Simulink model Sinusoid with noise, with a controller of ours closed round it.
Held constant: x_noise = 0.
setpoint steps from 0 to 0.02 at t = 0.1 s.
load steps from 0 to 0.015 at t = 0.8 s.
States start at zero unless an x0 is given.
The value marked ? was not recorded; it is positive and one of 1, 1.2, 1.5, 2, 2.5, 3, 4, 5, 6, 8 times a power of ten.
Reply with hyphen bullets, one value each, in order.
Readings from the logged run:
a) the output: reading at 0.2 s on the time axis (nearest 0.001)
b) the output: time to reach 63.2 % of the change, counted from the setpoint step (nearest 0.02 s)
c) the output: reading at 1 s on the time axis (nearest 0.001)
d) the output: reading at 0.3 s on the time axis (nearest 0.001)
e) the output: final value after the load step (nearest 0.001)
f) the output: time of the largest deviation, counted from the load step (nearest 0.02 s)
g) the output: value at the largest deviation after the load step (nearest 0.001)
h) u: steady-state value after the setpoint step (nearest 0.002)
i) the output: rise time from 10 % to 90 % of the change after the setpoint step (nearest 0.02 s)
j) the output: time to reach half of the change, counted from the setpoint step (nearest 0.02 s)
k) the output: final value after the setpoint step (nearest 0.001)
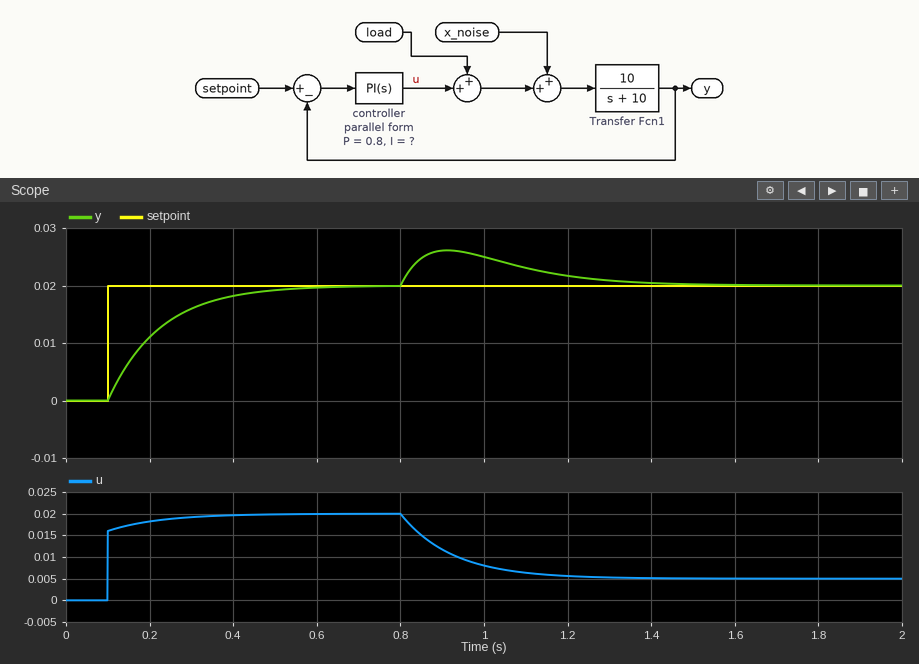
- 0.011
- 0.12 s
- 0.025
- 0.016
- 0.020
- 0.12 s
- 0.026
- 0.020
- 0.28 s
- 0.08 s
- 0.020
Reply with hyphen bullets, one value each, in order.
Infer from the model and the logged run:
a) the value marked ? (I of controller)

- 8
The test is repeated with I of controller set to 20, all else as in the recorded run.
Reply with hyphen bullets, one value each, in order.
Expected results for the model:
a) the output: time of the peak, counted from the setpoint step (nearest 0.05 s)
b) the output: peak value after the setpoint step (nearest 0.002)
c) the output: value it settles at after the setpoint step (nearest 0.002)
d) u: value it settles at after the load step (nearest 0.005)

- 0.25 s
- 0.022
- 0.020
- 0.005
